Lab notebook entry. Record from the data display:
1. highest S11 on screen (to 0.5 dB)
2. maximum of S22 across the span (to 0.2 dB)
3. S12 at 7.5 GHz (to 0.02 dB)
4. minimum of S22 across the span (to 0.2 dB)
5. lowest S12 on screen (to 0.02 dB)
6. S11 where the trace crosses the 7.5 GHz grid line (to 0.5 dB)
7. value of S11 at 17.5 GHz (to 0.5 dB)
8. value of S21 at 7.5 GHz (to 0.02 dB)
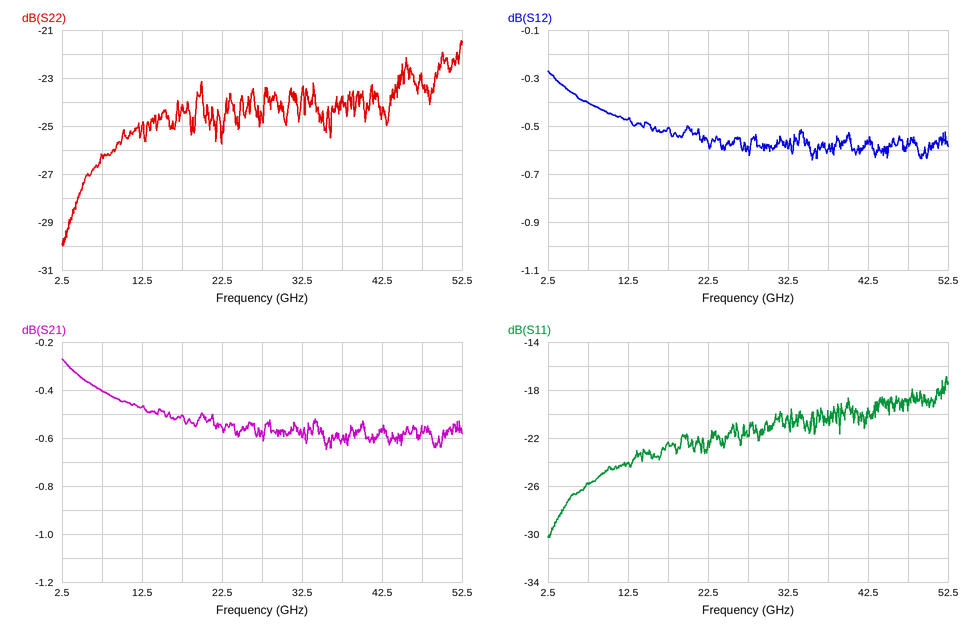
-17.0 dB
-21.4 dB
-0.40 dB
-30.0 dB
-0.64 dB
-26.0 dB
-22.5 dB
-0.40 dB
